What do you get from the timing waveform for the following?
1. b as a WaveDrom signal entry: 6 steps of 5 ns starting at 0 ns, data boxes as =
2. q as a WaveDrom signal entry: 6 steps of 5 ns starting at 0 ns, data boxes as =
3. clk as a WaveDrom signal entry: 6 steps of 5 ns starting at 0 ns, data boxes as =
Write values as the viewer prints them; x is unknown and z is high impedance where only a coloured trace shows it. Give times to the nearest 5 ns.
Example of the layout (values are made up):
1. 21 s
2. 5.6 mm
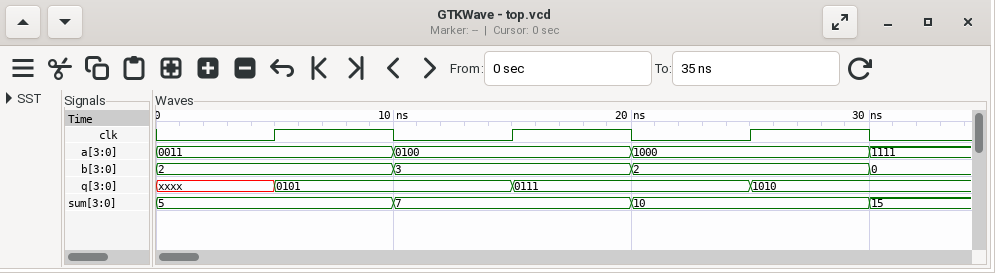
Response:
1. {name: 'b', wave: '=.=.=.', data: '2 3 2'}
2. {name: 'q', wave: 'x=.=.=', data: '0101 0111 1010'}
3. {name: 'clk', wave: '010101'}
